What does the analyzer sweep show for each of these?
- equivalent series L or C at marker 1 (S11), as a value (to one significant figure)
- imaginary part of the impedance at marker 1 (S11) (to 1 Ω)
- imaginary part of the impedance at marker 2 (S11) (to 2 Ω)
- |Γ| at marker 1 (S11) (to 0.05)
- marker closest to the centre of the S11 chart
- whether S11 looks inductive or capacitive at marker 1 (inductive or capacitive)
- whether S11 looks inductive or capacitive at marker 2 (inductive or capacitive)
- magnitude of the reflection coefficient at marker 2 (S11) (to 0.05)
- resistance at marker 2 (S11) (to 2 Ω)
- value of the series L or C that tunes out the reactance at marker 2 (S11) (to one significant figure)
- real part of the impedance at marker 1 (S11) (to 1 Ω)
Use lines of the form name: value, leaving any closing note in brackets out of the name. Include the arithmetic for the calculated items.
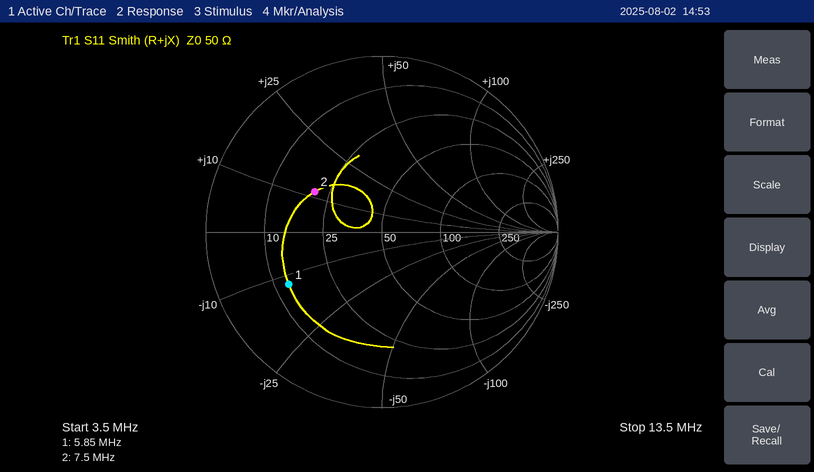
equivalent series L or C at marker 1 (S11), as a value: C = 1/(2π × 5.85 MHz × 12 Ω) ≈ 2 nF
imaginary part of the impedance at marker 1 (S11): -12 Ω
imaginary part of the impedance at marker 2 (S11): +12 Ω
|Γ| at marker 1 (S11): 0.60
marker closest to the centre of the S11 chart: marker 2
whether S11 looks inductive or capacitive at marker 1: capacitive
whether S11 looks inductive or capacitive at marker 2: inductive
magnitude of the reflection coefficient at marker 2 (S11): 0.45
resistance at marker 2 (S11): 20 Ω
value of the series L or C that tunes out the reactance at marker 2 (S11): C = 1/(2π × 7.5 MHz × 12 Ω) ≈ 2 nF
real part of the impedance at marker 1 (S11): 13 Ω
